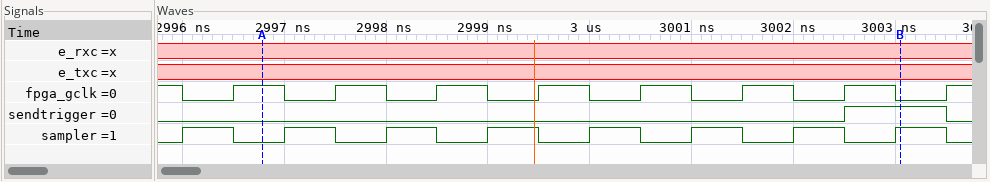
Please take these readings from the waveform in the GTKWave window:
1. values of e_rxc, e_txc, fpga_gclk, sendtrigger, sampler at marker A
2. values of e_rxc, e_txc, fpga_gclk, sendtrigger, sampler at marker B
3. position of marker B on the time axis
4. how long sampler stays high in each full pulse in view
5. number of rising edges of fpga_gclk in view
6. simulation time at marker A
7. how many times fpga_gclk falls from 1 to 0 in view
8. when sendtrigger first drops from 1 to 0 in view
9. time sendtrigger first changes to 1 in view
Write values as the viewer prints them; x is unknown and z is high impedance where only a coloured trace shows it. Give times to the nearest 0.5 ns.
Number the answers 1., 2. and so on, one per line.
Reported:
1. e_rxc=x, e_txc=x, fpga_gclk=1, sendtrigger=0, sampler=0
2. e_rxc=x, e_txc=x, fpga_gclk=0, sendtrigger=1, sampler=1
3. 3003 ns
4. 0.5 ns, 0.5 ns, 0.5 ns, 0.5 ns, 0.5 ns, 0.5 ns, 0.5 ns, 0.5 ns
5. 8
6. 2997 ns
7. 8
8. 3003.5 ns
9. 3002.5 ns
